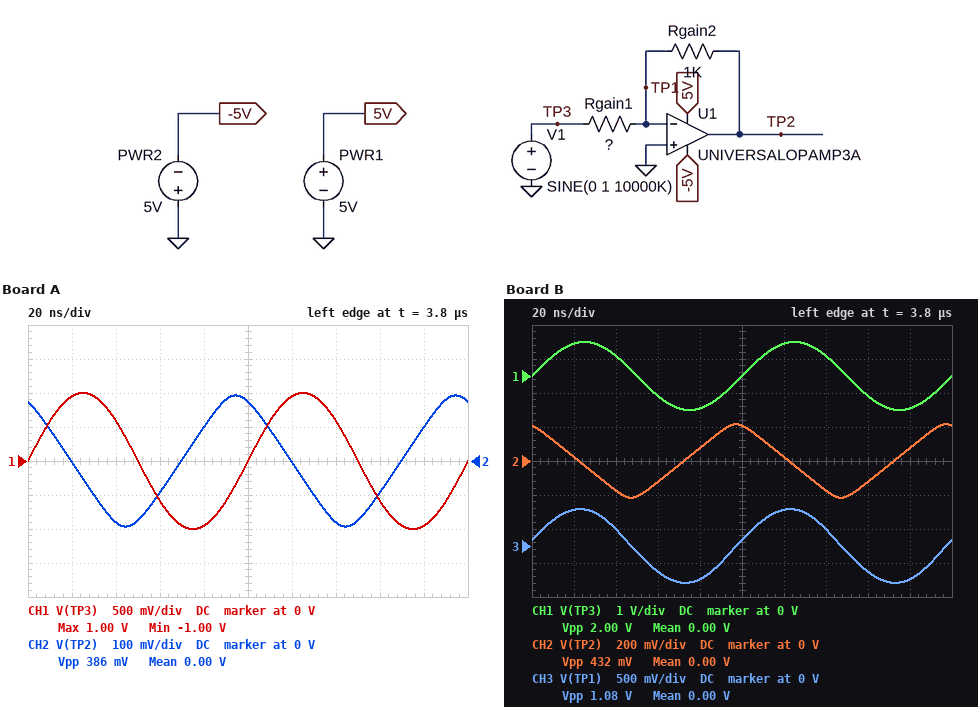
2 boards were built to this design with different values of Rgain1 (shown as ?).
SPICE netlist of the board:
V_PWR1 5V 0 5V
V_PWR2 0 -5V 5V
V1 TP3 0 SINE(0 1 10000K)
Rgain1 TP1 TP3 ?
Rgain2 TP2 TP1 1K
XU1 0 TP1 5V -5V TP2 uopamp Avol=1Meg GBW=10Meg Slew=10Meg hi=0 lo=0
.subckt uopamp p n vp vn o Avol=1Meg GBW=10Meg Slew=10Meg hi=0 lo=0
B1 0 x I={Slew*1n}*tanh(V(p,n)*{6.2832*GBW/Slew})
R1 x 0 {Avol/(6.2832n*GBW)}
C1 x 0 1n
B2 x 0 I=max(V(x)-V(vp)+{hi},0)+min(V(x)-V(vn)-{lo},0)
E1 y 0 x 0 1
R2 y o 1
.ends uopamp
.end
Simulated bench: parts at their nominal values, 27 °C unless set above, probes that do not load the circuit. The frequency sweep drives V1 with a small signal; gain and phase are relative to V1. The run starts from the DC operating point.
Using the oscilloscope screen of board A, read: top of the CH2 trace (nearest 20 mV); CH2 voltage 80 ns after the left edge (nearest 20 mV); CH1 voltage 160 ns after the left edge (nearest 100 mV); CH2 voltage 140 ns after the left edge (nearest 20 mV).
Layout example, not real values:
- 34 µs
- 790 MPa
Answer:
- 200 mV
- 100 mV
- -600 mV
- -180 mV
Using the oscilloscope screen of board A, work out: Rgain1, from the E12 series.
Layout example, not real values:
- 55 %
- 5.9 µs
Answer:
- 1.8 kΩ
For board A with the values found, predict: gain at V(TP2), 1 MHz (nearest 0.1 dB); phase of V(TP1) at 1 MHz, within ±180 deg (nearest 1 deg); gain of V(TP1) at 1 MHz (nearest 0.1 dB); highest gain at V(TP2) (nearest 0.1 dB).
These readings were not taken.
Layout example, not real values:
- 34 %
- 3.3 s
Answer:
- -5.2 dB
- 81 deg
- -25.2 dB
- -5.1 dB
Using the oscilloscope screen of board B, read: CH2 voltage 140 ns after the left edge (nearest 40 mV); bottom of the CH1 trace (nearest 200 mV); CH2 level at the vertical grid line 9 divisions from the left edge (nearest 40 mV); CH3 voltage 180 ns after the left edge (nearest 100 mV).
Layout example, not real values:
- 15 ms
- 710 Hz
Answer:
- -160 mV
- -1.0 V
- 80 mV
- -500 mV
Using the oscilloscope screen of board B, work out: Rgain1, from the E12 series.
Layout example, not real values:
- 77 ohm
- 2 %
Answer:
- 820 Ω
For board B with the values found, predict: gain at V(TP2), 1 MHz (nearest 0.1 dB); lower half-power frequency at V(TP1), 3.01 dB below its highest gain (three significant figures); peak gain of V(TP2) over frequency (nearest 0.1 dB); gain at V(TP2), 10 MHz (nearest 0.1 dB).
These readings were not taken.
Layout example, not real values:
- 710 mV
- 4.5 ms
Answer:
- 1.5 dB
- 4.50 MHz
- 1.7 dB
- -6.0 dB
